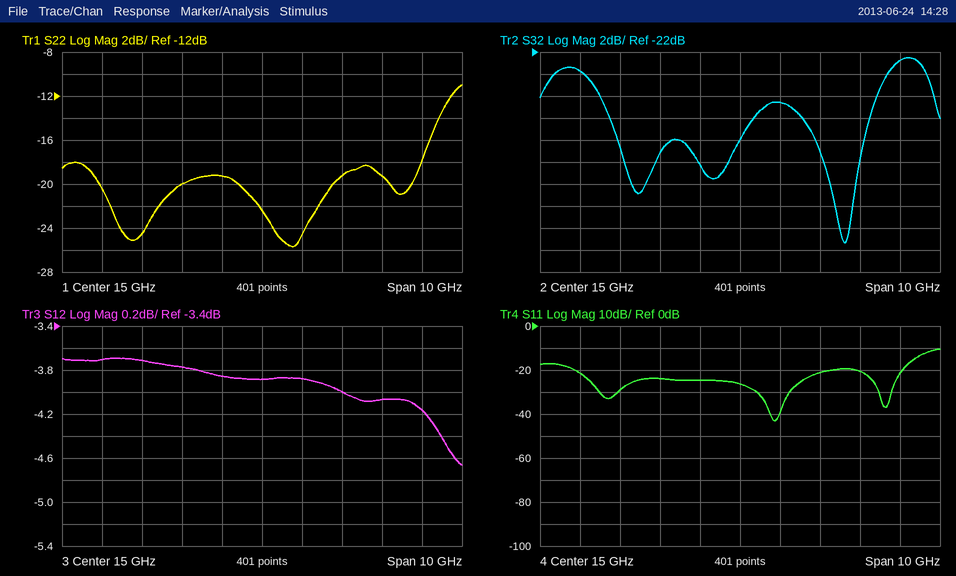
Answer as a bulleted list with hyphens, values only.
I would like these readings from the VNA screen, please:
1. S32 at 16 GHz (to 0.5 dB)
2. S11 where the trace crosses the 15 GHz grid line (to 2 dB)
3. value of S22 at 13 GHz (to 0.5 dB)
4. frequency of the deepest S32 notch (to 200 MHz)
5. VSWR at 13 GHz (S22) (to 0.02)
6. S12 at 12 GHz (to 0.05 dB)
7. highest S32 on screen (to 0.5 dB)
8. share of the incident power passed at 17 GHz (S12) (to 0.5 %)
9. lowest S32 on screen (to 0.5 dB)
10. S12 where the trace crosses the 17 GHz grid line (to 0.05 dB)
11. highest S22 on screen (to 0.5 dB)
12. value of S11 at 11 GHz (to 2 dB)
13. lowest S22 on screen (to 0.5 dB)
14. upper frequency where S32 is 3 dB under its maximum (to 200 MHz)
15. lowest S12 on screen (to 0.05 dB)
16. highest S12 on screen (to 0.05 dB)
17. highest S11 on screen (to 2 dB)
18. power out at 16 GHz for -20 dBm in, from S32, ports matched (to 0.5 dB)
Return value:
- -26.5 dB
- -26 dB
- -20.0 dB
- 17.6 GHz
- 1.22
- -3.70 dB
- -22.5 dB
- 40.0 %
- -39.5 dB
- -4.00 dB
- -11.0 dB
- -22 dB
- -25.5 dB
- 19.8 GHz
- -4.65 dB
- -3.70 dB
- -10 dB
- -46.5 dBm
